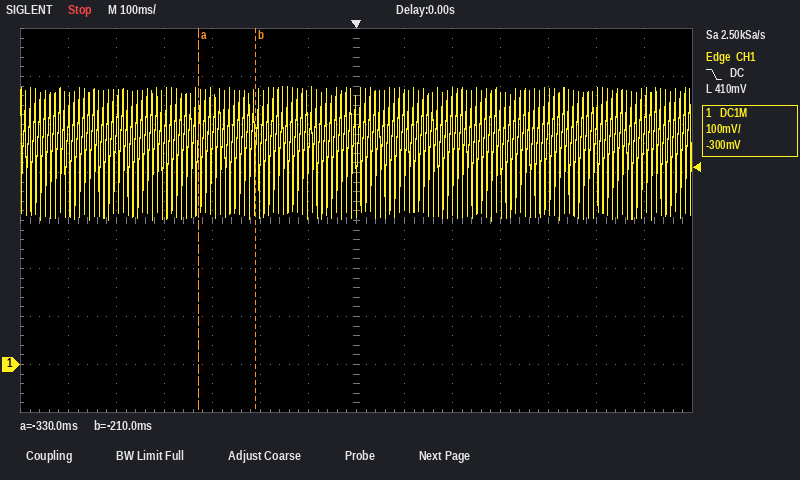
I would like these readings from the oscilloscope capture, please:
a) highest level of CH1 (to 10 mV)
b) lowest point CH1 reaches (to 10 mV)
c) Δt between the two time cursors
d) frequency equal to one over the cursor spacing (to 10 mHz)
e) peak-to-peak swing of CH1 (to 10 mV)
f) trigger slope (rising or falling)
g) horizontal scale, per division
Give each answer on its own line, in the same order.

580 mV
300 mV
120 ms
8.33 Hz
280 mV
falling
100 ms
